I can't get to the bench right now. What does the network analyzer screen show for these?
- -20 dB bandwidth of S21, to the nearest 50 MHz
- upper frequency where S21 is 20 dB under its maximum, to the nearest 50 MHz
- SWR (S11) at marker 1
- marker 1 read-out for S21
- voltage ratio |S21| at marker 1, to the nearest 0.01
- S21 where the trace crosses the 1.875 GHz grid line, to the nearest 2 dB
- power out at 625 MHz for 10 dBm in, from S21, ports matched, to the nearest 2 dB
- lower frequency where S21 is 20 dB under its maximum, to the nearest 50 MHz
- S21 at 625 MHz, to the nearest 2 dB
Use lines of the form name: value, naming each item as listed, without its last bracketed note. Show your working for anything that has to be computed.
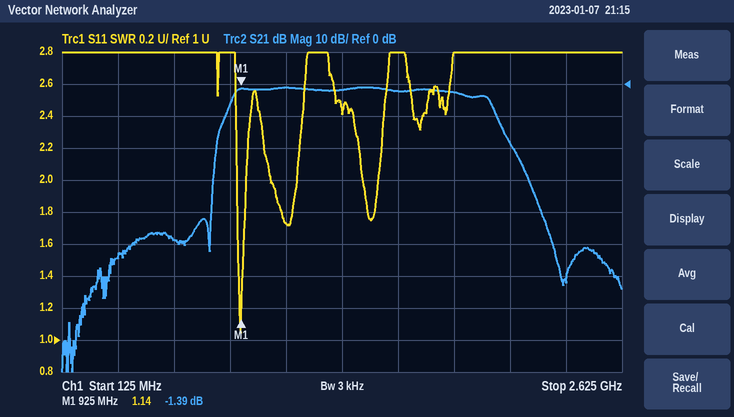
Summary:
-20 dB bandwidth of S21, to the nearest 50 MHz: 2.15 GHz − 800 MHz = 1.35 GHz
upper frequency where S21 is 20 dB under its maximum, to the nearest 50 MHz: 2.15 GHz
SWR (S11) at marker 1: 1.14
marker 1 read-out for S21: -1.39 dB
voltage ratio |S21| at marker 1, to the nearest 0.01: 10^(-1.39/20) ≈ 0.85
S21 where the trace crosses the 1.875 GHz grid line, to the nearest 2 dB: -2 dB
power out at 625 MHz for 10 dBm in, from S21, ports matched, to the nearest 2 dB: 10 dBm + (-48 dB) = -38 dBm
lower frequency where S21 is 20 dB under its maximum, to the nearest 50 MHz: 800 MHz
S21 at 625 MHz, to the nearest 2 dB: -48 dB
